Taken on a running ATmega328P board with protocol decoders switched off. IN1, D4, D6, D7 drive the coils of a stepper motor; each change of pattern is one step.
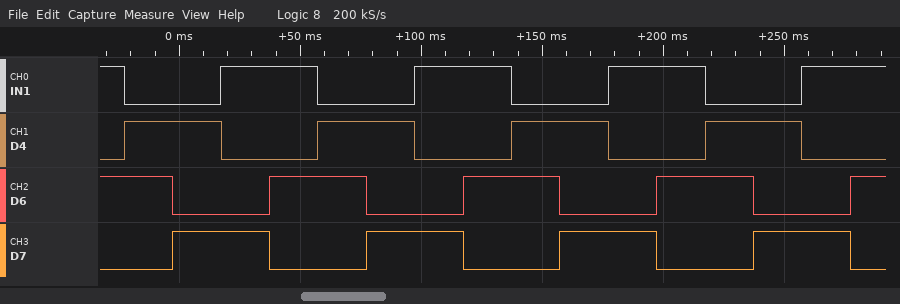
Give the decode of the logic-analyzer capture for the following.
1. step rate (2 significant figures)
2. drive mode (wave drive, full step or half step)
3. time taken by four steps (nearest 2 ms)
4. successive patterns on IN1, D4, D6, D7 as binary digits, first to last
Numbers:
50 steps/s
full step
80 ms
1010 0110 0101 1001 1010 0110 0101 1001 1010 0110 0101 1001 1010 0110 0101 1001 1010
